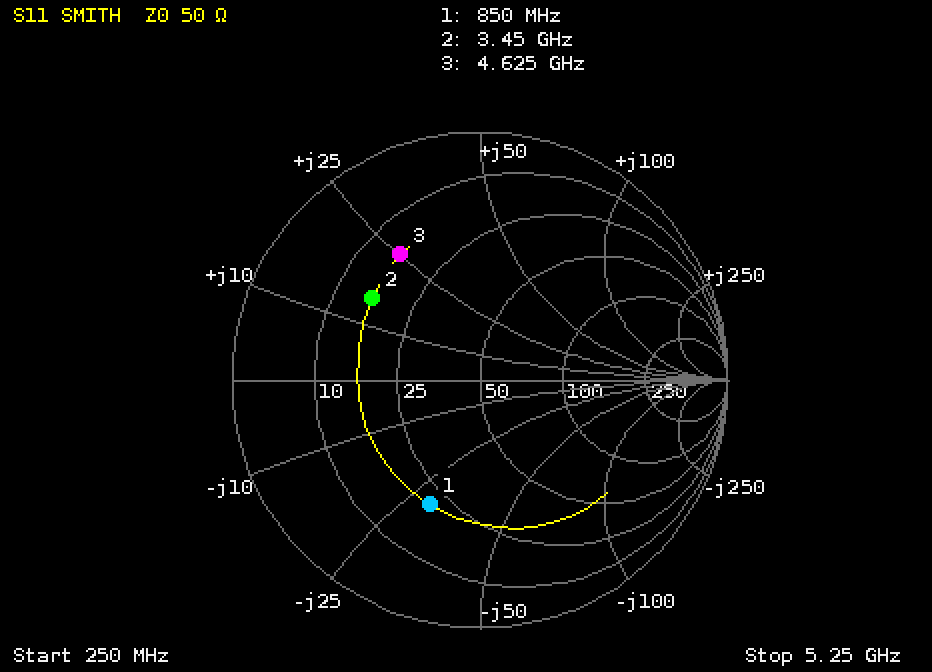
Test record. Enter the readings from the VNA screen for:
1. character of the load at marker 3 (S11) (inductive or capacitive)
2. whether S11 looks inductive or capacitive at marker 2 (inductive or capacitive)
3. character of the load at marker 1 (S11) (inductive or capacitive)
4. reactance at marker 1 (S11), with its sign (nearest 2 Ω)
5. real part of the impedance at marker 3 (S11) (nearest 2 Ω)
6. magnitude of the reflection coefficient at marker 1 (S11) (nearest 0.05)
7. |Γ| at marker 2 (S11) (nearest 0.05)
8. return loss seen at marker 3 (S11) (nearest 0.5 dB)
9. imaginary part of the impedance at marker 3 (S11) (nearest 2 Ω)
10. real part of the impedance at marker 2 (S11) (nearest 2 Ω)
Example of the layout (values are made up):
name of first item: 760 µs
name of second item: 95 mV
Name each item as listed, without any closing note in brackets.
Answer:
character of the load at marker 3 (S11): inductive
whether S11 looks inductive or capacitive at marker 2: inductive
character of the load at marker 1 (S11): capacitive
reactance at marker 1 (S11), with its sign: -30 Ω
real part of the impedance at marker 3 (S11): 16 Ω
magnitude of the reflection coefficient at marker 1 (S11): 0.55
|Γ| at marker 2 (S11): 0.55
return loss seen at marker 3 (S11): 4.5 dB
imaginary part of the impedance at marker 3 (S11): +26 Ω
real part of the impedance at marker 2 (S11): 16 Ω
